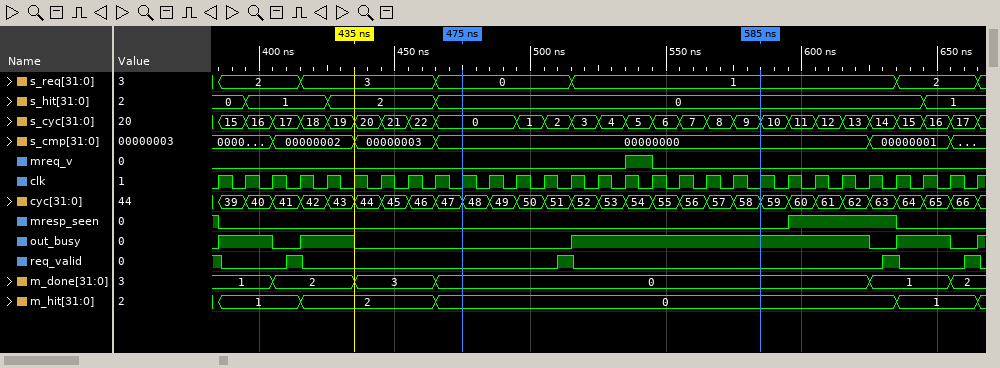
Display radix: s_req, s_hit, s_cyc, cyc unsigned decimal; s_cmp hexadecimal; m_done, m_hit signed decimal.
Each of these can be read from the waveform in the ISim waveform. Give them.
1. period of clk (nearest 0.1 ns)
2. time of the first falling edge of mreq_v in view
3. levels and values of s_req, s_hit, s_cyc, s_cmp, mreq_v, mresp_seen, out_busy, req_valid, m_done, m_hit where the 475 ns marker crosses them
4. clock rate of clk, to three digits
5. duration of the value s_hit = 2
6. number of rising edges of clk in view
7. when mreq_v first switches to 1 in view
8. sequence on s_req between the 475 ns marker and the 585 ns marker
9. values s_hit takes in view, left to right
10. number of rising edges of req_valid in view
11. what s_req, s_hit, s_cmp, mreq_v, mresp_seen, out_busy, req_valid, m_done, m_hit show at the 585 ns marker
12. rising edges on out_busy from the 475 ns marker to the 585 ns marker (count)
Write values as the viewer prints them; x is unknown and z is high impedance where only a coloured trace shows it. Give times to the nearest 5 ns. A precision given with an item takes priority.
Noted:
10 ns
545 ns
s_req=0, s_hit=0, s_cyc=0, s_cmp=00000000, mreq_v=0, mresp_seen=0, out_busy=0, req_valid=0, m_done=0, m_hit=0
100 MHz
40 ns
29
535 ns
0, 1
0, 1, 2, 0, 1
4
s_req=1, s_hit=0, s_cmp=00000000, mreq_v=0, mresp_seen=0, out_busy=1, req_valid=0, m_done=0, m_hit=0
1
